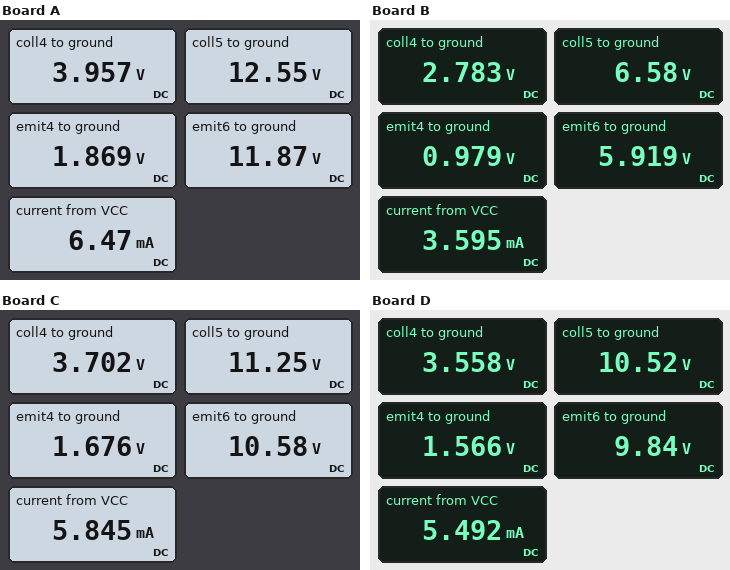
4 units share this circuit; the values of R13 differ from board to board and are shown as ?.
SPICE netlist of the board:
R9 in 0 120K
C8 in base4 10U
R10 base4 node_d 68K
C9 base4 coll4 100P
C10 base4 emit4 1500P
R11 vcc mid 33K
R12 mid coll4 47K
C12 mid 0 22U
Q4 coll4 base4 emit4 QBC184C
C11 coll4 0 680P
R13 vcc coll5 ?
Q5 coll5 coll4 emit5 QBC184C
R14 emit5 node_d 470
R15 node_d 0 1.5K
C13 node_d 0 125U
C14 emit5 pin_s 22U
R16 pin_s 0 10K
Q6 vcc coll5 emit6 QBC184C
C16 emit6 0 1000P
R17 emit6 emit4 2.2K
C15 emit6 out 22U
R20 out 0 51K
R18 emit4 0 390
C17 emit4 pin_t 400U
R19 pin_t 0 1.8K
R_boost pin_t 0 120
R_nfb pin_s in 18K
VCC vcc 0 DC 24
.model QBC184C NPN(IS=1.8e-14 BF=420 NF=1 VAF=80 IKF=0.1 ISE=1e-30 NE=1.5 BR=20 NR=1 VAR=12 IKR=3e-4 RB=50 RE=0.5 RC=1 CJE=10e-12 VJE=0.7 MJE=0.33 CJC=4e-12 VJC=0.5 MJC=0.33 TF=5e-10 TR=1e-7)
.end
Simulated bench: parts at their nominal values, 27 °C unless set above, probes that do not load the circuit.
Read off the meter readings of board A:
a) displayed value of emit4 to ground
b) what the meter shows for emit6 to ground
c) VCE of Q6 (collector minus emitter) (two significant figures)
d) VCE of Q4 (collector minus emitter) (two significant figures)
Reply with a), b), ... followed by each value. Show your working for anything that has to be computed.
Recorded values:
a) 1.869 V
b) 11.87 V
c) 24 V - 11.87 V = 12 V
d) 3.957 V - 1.869 V = 2.1 V
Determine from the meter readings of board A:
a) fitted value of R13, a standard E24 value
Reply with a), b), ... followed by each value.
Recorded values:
a) 6.8 kΩ
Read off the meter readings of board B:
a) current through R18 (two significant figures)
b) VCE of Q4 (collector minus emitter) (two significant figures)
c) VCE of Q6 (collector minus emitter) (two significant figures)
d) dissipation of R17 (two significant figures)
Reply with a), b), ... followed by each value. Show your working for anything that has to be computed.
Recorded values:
a) (979 mV) / 390 Ω = 2.5 mA
b) 2.783 V - 979 mV = 1.8 V
c) 24 V - 5.919 V = 18 V
d) (5.919 V - 979 mV)^2 / 2.2 kΩ = 11 mW
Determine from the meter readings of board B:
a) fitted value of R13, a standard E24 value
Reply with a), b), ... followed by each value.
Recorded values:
a) 16 kΩ
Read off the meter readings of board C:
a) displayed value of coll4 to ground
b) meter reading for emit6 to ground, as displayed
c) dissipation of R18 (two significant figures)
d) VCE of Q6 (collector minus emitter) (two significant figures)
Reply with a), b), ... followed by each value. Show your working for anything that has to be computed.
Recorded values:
a) 3.702 V
b) 10.58 V
c) (1.676 V)^2 / 390 Ω = 7.2 mW
d) 24 V - 10.58 V = 13 V
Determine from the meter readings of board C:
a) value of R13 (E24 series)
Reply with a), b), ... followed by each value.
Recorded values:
a) 8.2 kΩ
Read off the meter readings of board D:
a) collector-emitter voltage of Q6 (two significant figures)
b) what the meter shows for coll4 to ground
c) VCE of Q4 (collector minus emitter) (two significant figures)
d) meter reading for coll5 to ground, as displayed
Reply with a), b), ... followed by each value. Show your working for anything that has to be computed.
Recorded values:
a) 24 V - 9.84 V = 14 V
b) 3.558 V
c) 3.558 V - 1.566 V = 2.0 V
d) 10.52 V
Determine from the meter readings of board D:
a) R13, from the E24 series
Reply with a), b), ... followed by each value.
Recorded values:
a) 9.1 kΩ
